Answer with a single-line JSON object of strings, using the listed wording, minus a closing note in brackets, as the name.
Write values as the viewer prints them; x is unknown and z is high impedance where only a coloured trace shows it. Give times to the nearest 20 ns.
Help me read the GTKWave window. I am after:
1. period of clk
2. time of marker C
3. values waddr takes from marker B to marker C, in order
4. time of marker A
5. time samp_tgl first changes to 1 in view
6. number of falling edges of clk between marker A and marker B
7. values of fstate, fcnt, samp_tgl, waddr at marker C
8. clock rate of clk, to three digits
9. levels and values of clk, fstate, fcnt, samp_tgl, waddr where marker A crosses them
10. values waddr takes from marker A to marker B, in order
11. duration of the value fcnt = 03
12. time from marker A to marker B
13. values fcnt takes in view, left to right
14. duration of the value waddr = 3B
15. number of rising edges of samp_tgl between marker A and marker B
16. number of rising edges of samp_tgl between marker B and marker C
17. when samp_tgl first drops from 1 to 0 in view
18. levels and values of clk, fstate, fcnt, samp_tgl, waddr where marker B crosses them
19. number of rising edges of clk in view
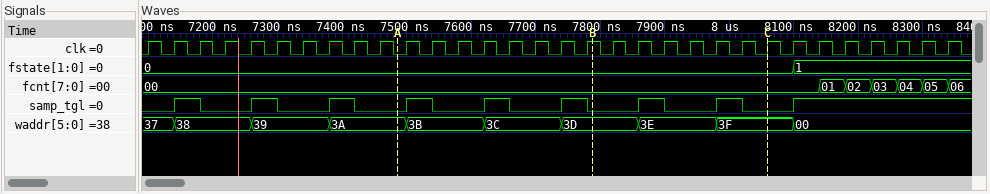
{"period of clk": "40 ns", "time of marker C": "8060 ns", "values waddr takes from marker B to marker C, in order": "3D, 3E, 3F", "time of marker A": "7480 ns", "time samp_tgl first changes to 1 in view": "7140 ns", "number of falling edges of clk between marker A and marker B": "7", "values of fstate, fcnt, samp_tgl, waddr at marker C": "fstate=0, fcnt=00, samp_tgl=0, waddr=3F", "clock rate of clk, to three digits": "25.0 MHz", "levels and values of clk, fstate, fcnt, samp_tgl, waddr where marker A crosses them": "clk=0, fstate=0, fcnt=00, samp_tgl=0, waddr=3A", "values waddr takes from marker A to marker B, in order": "3A, 3B, 3C, 3D", "duration of the value fcnt = 03": "40 ns", "time from marker A to marker B": "300 ns", "values fcnt takes in view, left to right": "00, 01, 02, 03, 04, 05, 06", "duration of the value waddr = 3B": "120 ns", "number of rising edges of samp_tgl between marker A and marker B": "3", "number of rising edges of samp_tgl between marker B and marker C": "2", "when samp_tgl first drops from 1 to 0 in view": "7180 ns", "levels and values of clk, fstate, fcnt, samp_tgl, waddr where marker B crosses them": "clk=1, fstate=0, fcnt=00, samp_tgl=0, waddr=3D", "number of rising edges of clk in view": "32"}
